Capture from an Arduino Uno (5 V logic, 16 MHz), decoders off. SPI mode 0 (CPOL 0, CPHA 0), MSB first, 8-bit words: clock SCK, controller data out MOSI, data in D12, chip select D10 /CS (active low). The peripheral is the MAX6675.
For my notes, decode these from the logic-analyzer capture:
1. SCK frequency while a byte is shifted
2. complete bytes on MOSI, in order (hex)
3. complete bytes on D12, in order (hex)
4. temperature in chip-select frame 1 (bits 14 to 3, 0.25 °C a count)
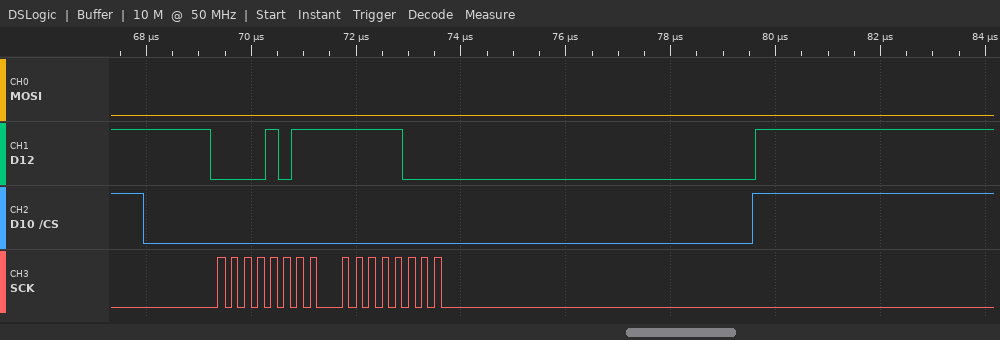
4 MHz
00 00
0B F8
95.75 °C
